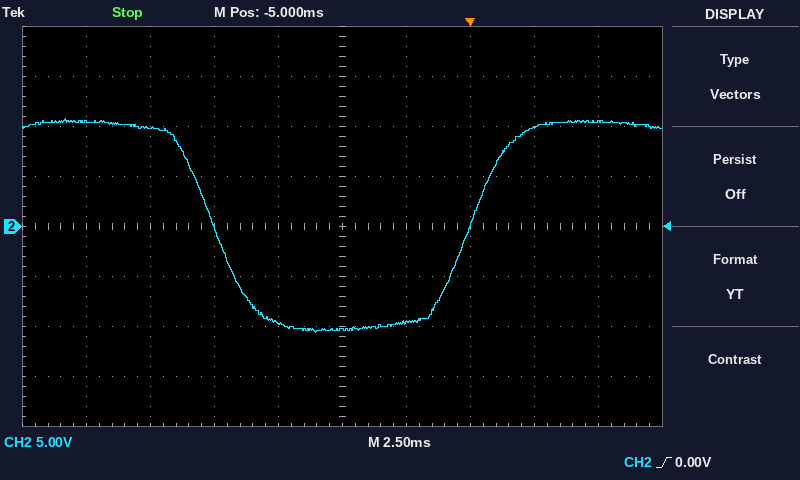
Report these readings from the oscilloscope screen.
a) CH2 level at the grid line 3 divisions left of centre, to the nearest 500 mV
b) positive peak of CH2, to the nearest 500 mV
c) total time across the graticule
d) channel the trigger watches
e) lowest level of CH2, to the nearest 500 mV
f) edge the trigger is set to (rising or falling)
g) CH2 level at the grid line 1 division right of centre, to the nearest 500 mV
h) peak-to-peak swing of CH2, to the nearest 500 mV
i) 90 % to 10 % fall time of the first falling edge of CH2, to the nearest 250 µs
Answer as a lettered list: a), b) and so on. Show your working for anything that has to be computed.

a) 10.0 V
b) 11.0 V
c) 25 ms
d) CH2
e) -10.5 V
f) rising
g) -9.5 V
h) 11.0 V − (-10.5 V) = 21.5 V
i) 3.00 ms
